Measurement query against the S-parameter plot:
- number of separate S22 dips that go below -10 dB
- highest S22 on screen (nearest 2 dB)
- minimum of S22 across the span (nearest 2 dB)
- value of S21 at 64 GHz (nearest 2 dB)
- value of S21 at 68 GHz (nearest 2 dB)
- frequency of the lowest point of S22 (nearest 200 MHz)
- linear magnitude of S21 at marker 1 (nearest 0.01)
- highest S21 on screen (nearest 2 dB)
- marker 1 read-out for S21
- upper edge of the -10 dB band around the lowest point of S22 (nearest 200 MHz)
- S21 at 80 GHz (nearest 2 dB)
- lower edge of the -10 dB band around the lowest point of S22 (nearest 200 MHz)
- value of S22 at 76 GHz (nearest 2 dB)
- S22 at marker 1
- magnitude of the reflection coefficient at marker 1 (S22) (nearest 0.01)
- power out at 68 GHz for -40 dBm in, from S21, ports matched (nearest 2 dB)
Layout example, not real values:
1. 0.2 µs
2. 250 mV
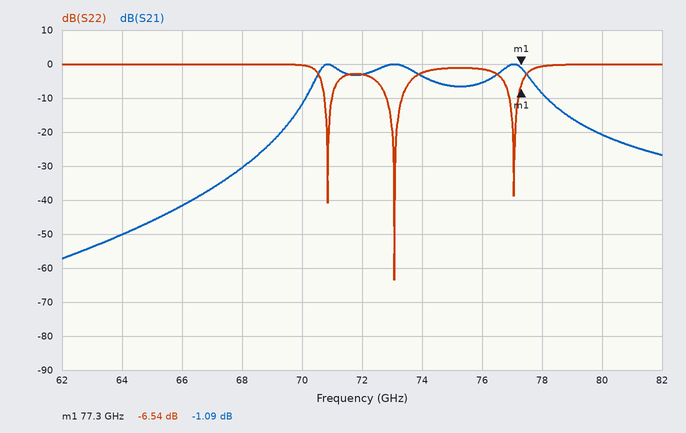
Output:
1. 3
2. 0 dB
3. -64 dB
4. -50 dB
5. -30 dB
6. 73.0 GHz
7. 0.88
8. 0 dB
9. -1.09 dB
10. 73.4 GHz
11. -20 dB
12. 72.8 GHz
13. -2 dB
14. -6.54 dB
15. 0.47
16. -70 dBm
